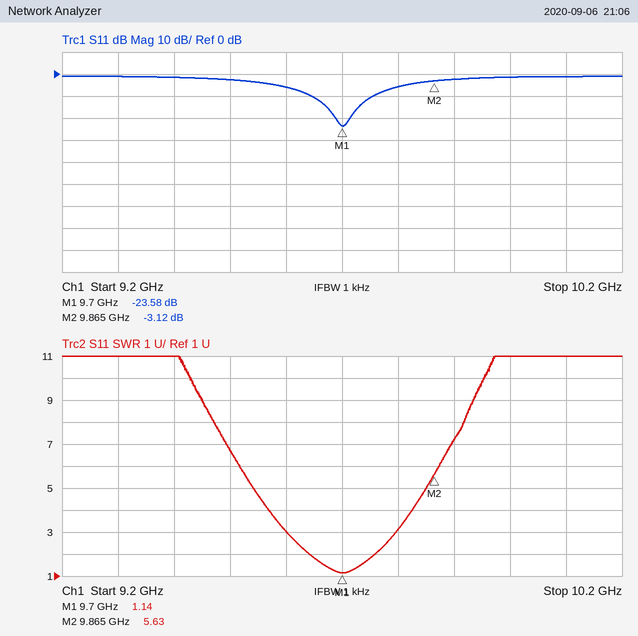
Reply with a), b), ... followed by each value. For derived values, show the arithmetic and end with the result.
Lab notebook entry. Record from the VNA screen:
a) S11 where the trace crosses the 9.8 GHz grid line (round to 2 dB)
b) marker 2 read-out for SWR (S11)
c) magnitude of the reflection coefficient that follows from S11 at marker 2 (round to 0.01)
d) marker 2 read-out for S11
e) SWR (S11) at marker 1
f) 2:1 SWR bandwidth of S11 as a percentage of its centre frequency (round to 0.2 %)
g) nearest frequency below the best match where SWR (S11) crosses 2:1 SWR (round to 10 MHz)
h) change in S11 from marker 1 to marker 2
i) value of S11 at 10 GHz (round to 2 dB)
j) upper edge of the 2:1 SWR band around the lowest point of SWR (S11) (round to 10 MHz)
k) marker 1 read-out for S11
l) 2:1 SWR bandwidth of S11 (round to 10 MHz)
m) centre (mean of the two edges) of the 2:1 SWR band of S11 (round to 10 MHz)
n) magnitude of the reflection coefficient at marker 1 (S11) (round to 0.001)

a) -6 dB
b) 5.63
c) 10^(-3.12/20) ≈ 0.70
d) -3.12 dB
e) 1.14
f) 120 MHz / 9.7 GHz ≈ 1.2 %
g) 9.64 GHz
h) -3.12 − (-23.58) = 20.46 dB
i) -2 dB
j) 9.76 GHz
k) -23.58 dB
l) 9.76 GHz − 9.64 GHz = 120 MHz
m) 9.70 GHz
n) 10^(-23.58/20) ≈ 0.066
